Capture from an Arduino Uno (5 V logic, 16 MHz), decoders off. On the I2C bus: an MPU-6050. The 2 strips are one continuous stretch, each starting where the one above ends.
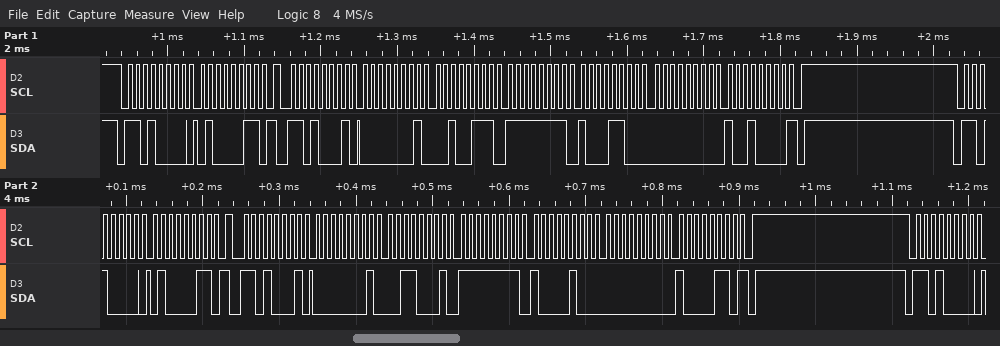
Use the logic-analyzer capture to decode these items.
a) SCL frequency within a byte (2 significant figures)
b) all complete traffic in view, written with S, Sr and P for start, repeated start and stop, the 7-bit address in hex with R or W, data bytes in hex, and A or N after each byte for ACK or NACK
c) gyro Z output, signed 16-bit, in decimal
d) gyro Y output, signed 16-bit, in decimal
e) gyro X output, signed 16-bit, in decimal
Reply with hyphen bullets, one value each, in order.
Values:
- 100 kHz
- S 68W A 43 A Sr 68R A 01 A 27 A FF A 8C A 00 A 90 N P S 68W A 43 A Sr 68R A 01 A 31 A FF A 84 A 00 A 86 N P S 68W A
- 144
- -116
- 295
